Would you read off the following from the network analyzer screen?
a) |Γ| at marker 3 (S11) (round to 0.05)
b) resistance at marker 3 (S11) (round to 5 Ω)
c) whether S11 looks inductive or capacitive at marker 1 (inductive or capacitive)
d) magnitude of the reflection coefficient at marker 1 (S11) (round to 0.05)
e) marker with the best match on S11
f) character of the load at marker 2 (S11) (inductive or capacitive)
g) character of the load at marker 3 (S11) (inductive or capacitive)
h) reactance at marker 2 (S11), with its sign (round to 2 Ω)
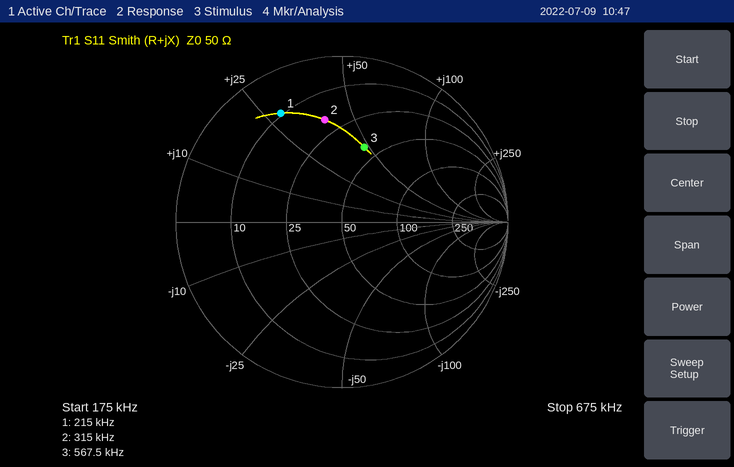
0.45
40 Ω
inductive
0.75
marker 3
inductive
inductive
+38 Ω
